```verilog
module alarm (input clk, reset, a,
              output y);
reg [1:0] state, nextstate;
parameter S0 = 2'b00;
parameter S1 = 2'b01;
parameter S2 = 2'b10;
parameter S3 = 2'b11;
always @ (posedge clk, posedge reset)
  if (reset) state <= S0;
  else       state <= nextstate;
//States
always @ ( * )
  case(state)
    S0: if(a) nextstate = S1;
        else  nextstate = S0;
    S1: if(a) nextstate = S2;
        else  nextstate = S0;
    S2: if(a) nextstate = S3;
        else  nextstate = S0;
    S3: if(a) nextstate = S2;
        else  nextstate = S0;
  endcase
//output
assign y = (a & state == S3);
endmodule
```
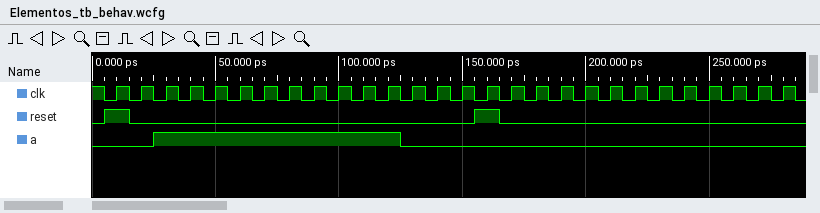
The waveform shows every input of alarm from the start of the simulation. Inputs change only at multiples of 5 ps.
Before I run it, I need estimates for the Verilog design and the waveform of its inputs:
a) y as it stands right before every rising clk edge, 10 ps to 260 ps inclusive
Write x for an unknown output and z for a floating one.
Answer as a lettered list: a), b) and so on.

a) 0 0 0 0 0 1 0 1 0 1 0 1 0 0 0 0 0 0 0 0 0 0 0 0 0 0
